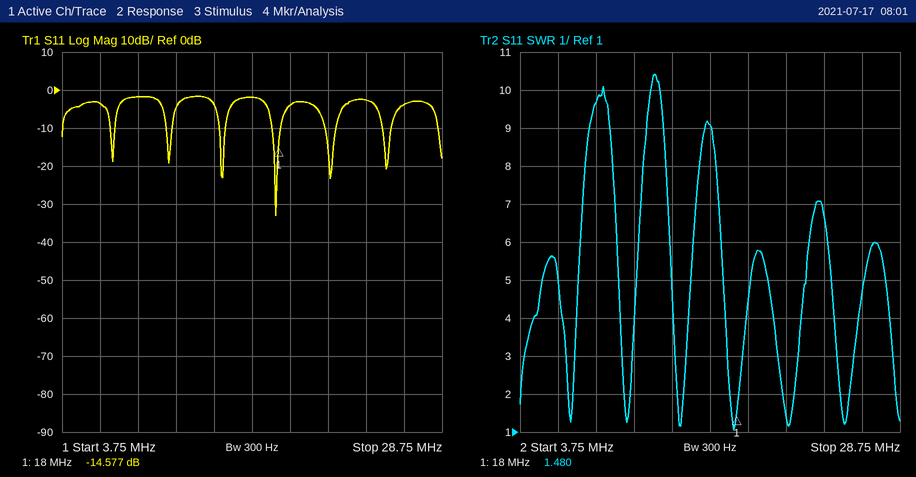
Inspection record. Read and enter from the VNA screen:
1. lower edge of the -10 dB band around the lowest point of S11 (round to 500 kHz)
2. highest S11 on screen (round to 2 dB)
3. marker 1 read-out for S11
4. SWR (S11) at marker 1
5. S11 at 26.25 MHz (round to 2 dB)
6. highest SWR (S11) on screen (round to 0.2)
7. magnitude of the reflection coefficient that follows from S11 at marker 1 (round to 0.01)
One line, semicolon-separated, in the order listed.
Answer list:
17.5 MHz; -2 dB; -14.577 dB; 1.480; -4 dB; 10.4; 0.19
